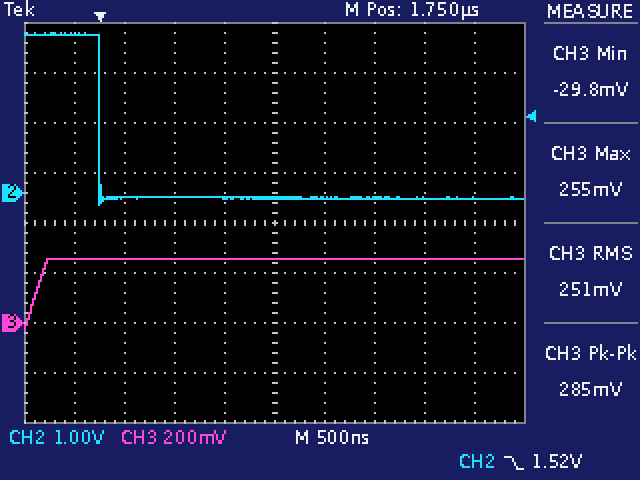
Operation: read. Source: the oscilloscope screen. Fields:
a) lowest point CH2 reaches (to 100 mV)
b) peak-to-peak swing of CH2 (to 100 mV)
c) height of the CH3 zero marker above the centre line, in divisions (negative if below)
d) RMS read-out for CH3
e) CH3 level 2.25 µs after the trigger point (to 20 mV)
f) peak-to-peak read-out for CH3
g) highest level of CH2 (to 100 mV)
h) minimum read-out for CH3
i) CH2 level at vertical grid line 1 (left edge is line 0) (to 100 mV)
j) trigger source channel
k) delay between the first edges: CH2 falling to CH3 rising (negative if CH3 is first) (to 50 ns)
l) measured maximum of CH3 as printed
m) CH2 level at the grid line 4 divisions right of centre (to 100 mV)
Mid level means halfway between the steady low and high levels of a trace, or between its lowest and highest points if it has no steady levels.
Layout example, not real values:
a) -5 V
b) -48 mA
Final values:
a) -200 mV
b) 3.4 V
c) -2.0 div
d) 251 mV
e) 260 mV
f) 285 mV
g) 3.2 V
h) -29.8 mV
i) 3.2 V
j) CH2
k) -650 ns
l) 255 mV
m) -100 mV
